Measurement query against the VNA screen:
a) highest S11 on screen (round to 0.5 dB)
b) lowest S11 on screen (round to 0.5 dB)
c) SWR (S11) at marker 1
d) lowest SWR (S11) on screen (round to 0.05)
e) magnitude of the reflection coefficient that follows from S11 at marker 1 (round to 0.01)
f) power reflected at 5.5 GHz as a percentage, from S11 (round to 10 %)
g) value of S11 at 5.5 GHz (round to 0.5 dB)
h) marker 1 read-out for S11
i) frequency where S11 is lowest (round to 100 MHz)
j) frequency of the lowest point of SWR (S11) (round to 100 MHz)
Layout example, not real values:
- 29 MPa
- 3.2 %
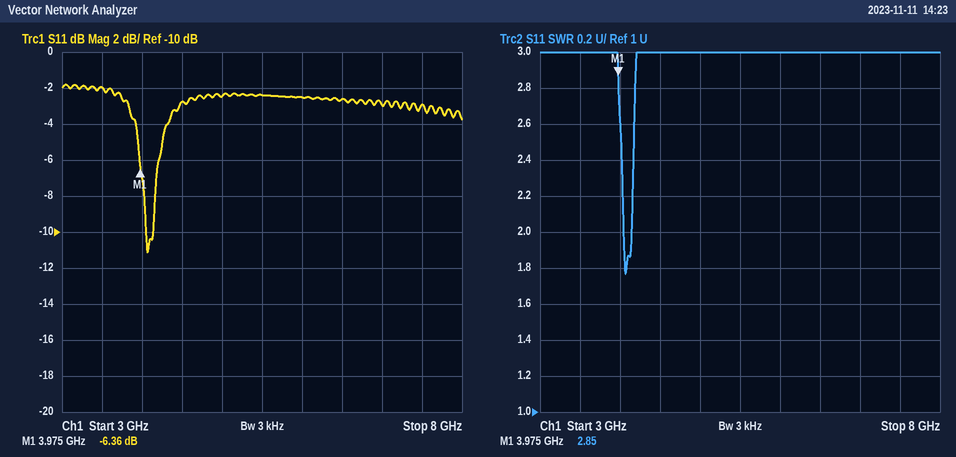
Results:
- -2.0 dB
- -11.0 dB
- 2.85
- 1.75
- 0.48
- 60 %
- -2.5 dB
- -6.36 dB
- 4.1 GHz
- 4.1 GHz
